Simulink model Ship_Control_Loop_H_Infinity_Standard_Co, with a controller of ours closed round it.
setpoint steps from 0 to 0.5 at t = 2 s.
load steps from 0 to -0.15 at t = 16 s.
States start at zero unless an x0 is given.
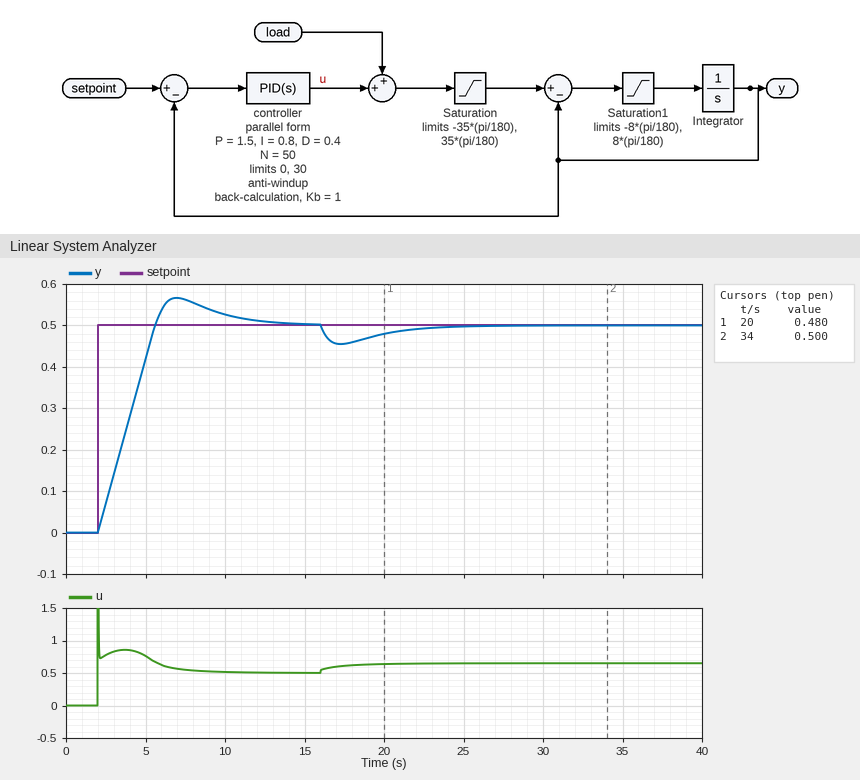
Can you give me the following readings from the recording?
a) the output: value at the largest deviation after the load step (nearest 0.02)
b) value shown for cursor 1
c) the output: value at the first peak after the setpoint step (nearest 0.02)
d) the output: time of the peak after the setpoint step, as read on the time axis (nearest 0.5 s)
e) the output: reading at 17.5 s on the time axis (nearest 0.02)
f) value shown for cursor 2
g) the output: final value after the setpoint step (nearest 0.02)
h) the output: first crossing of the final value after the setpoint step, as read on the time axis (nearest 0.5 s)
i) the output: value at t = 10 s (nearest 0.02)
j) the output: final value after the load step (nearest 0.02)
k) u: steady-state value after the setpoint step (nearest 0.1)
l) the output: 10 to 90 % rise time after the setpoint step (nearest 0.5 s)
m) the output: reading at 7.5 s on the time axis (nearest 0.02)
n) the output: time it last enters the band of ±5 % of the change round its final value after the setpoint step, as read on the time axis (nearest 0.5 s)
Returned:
0.46
0.480
0.56
7.0 s
0.46
0.500
0.50
5.5 s
0.52
0.50
0.5
3.0 s
0.56
10.0 s
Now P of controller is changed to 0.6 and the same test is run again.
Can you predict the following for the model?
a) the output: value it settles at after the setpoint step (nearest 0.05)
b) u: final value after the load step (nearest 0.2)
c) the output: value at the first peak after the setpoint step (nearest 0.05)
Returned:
0.50
0.6
0.60
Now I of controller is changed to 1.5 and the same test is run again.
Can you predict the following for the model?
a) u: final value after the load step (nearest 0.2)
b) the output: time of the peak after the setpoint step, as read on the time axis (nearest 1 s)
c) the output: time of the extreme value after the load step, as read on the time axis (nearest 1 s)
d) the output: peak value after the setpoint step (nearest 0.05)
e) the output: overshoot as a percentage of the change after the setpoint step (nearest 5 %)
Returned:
0.6
10 s
17 s
0.60
20 %
